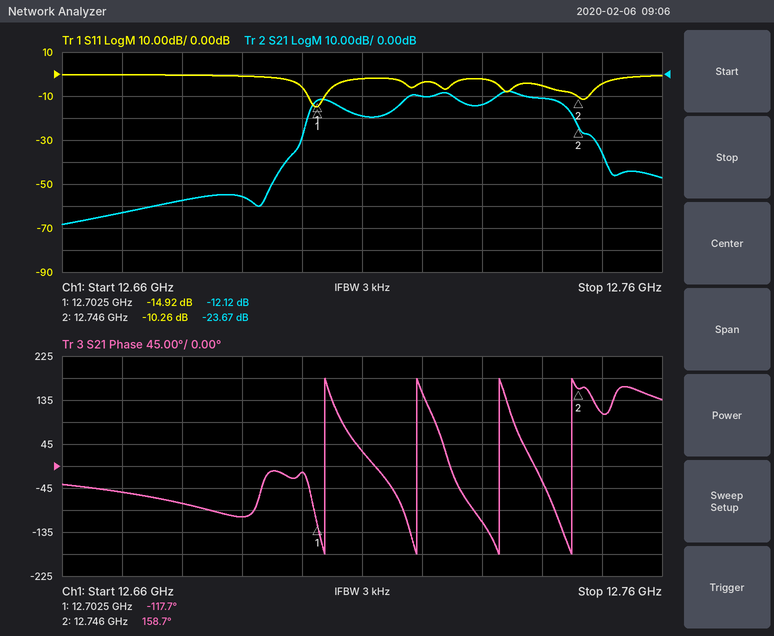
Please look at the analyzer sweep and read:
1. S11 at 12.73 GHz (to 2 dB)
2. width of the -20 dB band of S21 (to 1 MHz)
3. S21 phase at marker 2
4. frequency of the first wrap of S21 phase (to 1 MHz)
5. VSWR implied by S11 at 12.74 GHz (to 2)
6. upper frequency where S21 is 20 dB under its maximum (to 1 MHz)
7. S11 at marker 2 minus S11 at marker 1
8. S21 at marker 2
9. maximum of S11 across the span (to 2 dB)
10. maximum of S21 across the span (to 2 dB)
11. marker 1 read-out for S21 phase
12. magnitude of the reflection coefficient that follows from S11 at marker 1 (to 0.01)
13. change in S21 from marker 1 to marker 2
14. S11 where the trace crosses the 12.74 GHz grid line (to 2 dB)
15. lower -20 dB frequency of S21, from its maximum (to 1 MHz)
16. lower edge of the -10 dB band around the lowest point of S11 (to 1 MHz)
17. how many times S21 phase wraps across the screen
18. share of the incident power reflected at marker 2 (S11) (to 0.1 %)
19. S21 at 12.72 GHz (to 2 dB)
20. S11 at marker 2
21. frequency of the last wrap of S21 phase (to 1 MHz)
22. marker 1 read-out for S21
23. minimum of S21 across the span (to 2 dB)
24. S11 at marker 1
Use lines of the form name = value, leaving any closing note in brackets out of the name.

S11 at 12.73 GHz = -2 dB
width of the -20 dB band of S21 = 48 MHz
S21 phase at marker 2 = 158.7°
frequency of the first wrap of S21 phase = 12.704 GHz
VSWR implied by S11 at 12.74 GHz = 4
upper frequency where S21 is 20 dB under its maximum = 12.748 GHz
S11 at marker 2 minus S11 at marker 1 = 4.66 dB
S21 at marker 2 = -23.67 dB
maximum of S11 across the span = 0 dB
maximum of S21 across the span = -8 dB
marker 1 read-out for S21 phase = -117.7°
magnitude of the reflection coefficient that follows from S11 at marker 1 = 0.18
change in S21 from marker 1 to marker 2 = -11.55 dB
S11 where the trace crosses the 12.74 GHz grid line = -6 dB
lower -20 dB frequency of S21, from its maximum = 12.700 GHz
lower edge of the -10 dB band around the lowest point of S11 = 12.701 GHz
how many times S21 phase wraps across the screen = 4
share of the incident power reflected at marker 2 (S11) = 9.4 %
S21 at 12.72 GHz = -10 dB
S11 at marker 2 = -10.26 dB
frequency of the last wrap of S21 phase = 12.745 GHz
marker 1 read-out for S21 = -12.12 dB
minimum of S21 across the span = -68 dB
S11 at marker 1 = -14.92 dB
